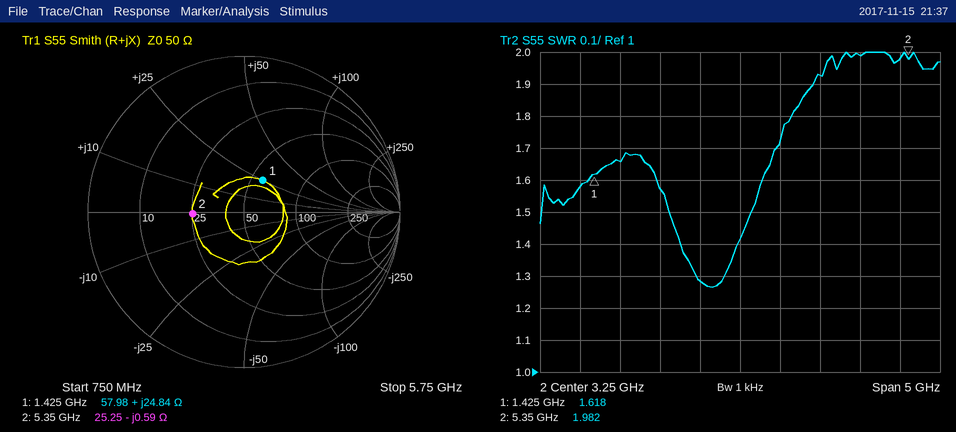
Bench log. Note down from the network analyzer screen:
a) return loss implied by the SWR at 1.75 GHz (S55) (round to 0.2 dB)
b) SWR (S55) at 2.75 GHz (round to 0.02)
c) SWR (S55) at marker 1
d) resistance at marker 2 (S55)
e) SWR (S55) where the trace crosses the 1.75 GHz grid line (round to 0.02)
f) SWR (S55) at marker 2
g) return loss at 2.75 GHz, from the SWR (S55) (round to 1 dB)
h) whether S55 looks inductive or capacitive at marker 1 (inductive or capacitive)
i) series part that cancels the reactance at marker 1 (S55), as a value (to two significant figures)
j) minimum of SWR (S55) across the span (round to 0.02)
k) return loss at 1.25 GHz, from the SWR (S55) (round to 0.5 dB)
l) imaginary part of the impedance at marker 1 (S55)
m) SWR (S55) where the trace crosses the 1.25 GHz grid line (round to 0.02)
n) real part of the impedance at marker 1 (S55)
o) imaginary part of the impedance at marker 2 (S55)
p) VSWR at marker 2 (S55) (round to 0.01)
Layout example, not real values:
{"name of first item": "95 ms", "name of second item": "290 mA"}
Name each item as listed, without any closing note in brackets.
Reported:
{"return loss implied by the SWR at 1.75 GHz (S55)": "12.2 dB", "SWR (S55) at 2.75 GHz": "1.28", "SWR (S55) at marker 1": "1.618", "resistance at marker 2": "25.25 Ω", "SWR (S55) where the trace crosses the 1.75 GHz grid line": "1.66", "SWR (S55) at marker 2": "1.982", "return loss at 2.75 GHz, from the SWR (S55)": "18 dB", "whether S55 looks inductive or capacitive at marker 1": "inductive", "series part that cancels the reactance at marker 1 (S55), as a value": "4.5 pF", "minimum of SWR (S55) across the span": "1.26", "return loss at 1.25 GHz, from the SWR (S55)": "13.0 dB", "imaginary part of the impedance at marker 1": "+24.84 Ω", "SWR (S55) where the trace crosses the 1.25 GHz grid line": "1.58", "real part of the impedance at marker 1": "57.98 Ω", "imaginary part of the impedance at marker 2": "-0.59 Ω", "VSWR at marker 2 (S55)": "1.98"}
